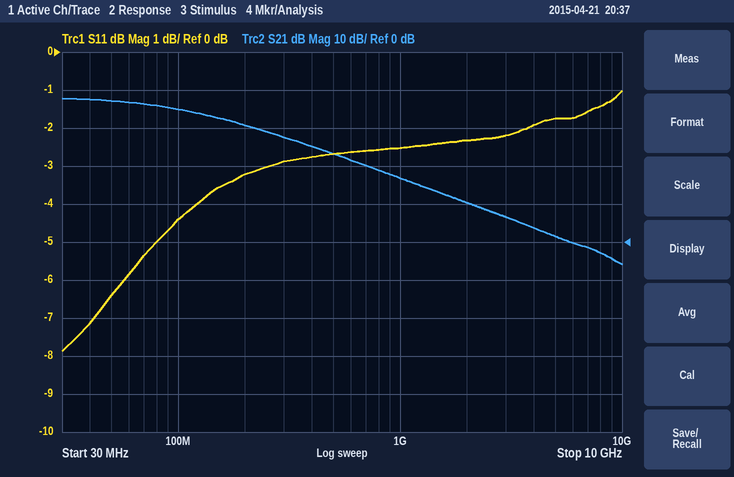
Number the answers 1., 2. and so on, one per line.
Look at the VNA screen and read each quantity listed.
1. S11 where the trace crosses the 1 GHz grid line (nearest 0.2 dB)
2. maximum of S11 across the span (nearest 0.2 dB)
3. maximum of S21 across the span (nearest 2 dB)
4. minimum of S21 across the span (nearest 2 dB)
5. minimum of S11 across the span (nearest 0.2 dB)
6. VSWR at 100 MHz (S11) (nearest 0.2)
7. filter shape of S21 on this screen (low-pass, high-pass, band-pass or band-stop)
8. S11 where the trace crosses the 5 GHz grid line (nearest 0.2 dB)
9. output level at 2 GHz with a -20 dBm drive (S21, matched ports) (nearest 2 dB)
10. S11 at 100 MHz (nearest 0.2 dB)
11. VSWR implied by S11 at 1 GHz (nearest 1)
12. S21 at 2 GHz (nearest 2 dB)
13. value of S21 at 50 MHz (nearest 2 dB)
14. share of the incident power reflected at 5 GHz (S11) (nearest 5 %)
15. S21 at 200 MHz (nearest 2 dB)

1. -2.6 dB
2. -1.0 dB
3. 38 dB
4. -6 dB
5. -7.8 dB
6. 4.0
7. low-pass
8. -1.8 dB
9. -10 dBm
10. -4.4 dB
11. 7
12. 10 dB
13. 38 dB
14. 65 %
15. 30 dB
